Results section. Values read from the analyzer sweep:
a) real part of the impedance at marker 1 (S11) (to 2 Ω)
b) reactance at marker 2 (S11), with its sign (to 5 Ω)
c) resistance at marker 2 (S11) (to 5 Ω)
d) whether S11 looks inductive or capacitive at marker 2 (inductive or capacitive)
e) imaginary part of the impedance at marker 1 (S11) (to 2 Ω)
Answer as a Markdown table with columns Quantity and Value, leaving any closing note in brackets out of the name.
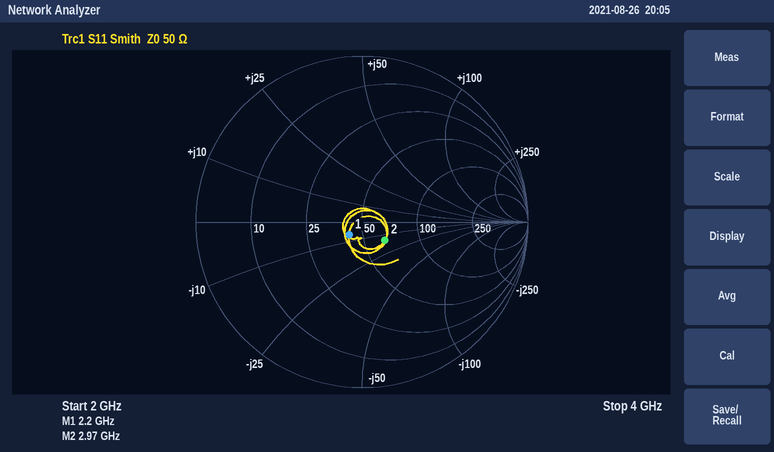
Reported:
| Quantity | Value |
|---|---|
| real part of the impedance at marker 1 (S11) | 42 Ω |
| reactance at marker 2 (S11), with its sign | -15 Ω |
| resistance at marker 2 (S11) | 65 Ω |
| whether S11 looks inductive or capacitive at marker 2 | capacitive |
| imaginary part of the impedance at marker 1 (S11) | -6 Ω |
